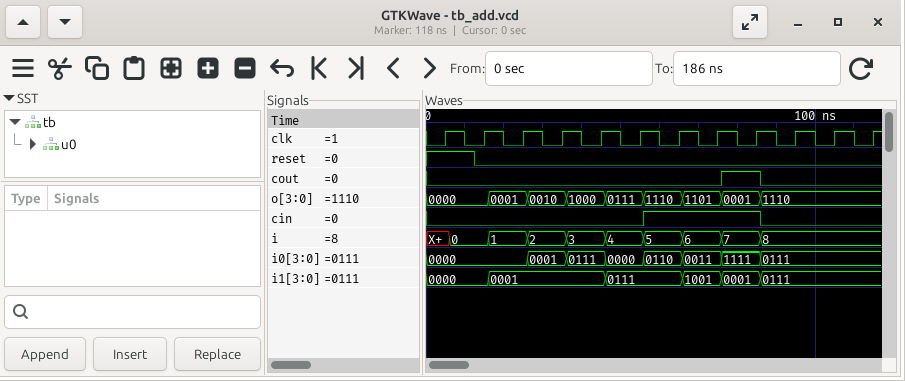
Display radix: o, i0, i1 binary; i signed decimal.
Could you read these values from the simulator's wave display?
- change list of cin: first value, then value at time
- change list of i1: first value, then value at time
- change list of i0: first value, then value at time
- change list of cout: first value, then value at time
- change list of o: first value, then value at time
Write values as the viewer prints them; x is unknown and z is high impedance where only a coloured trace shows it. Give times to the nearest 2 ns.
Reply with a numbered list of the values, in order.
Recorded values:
1. 0, 1 at 56 ns, 0 at 86 ns
2. 0000, 0001 at 16 ns, 0111 at 46 ns, 1001 at 66 ns, 0001 at 76 ns, 0111 at 86 ns
3. 0000, 0001 at 26 ns, 0111 at 36 ns, 0000 at 46 ns, 0110 at 56 ns, 0011 at 66 ns, 1111 at 76 ns, 0111 at 86 ns
4. 0, 1 at 76 ns, 0 at 86 ns
5. 0000, 0001 at 16 ns, 0010 at 26 ns, 1000 at 36 ns, 0111 at 46 ns, 1110 at 56 ns, 1101 at 66 ns, 0001 at 76 ns, 1110 at 86 ns
